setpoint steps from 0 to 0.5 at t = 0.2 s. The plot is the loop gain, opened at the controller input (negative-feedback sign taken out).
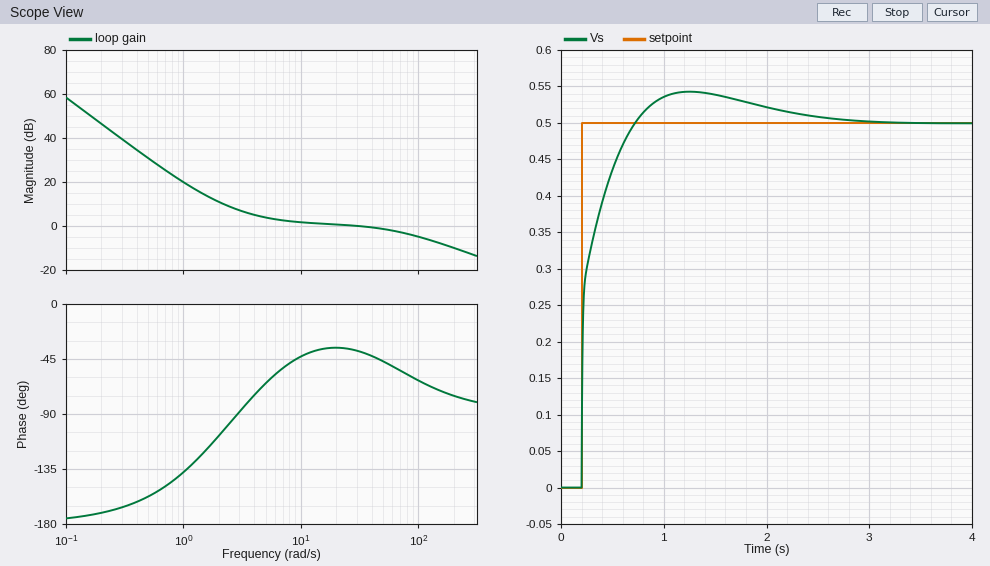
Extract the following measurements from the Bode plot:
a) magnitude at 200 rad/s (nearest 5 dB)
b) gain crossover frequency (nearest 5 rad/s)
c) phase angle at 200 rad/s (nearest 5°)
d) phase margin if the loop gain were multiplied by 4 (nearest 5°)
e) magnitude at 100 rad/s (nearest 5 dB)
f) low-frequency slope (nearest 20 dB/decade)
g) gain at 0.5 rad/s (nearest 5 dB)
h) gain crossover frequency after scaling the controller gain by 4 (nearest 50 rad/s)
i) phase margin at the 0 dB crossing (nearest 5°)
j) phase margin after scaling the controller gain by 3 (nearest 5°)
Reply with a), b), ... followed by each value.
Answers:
a) -10 dB
b) 30 rad/s
c) -75°
d) 100°
e) -5 dB
f) -40 dB/decade
g) 30 dB
h) 250 rad/s
i) 140°
j) 105°
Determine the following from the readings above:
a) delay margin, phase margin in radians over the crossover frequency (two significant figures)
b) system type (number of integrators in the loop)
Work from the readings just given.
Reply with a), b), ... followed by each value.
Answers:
a) 0.081 s
b) 2
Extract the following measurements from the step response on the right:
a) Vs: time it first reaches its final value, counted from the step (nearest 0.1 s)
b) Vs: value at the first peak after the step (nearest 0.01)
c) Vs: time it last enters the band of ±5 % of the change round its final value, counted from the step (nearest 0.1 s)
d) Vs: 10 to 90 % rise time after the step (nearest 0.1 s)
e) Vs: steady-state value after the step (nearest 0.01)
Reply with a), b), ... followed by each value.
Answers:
a) 0.5 s
b) 0.54
c) 1.7 s
d) 0.3 s
e) 0.50
